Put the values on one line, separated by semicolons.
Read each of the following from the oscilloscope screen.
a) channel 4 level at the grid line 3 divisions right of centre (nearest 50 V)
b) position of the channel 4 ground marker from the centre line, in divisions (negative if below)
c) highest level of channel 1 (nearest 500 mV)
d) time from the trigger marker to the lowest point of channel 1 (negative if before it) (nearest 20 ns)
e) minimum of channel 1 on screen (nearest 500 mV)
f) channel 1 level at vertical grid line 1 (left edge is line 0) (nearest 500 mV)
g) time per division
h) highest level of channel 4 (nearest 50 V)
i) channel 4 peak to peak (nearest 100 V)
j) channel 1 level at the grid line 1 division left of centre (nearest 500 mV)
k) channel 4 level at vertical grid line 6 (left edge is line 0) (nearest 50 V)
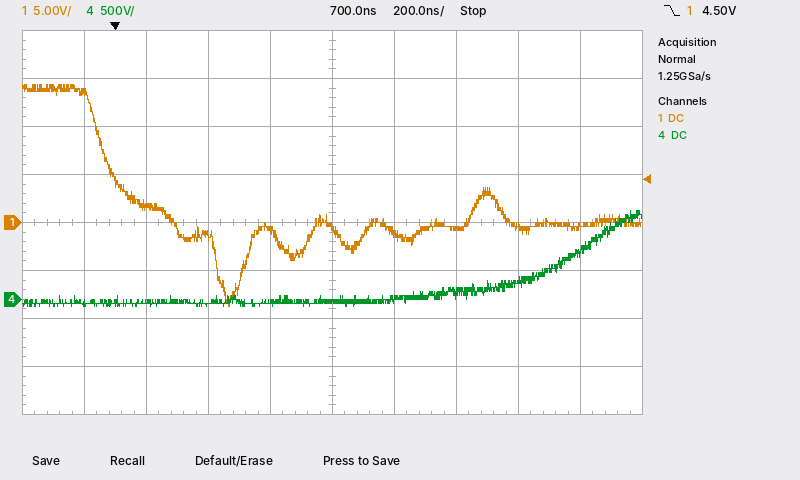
200 V; -1.6 div; 14.5 V; +360 ns; -9.0 V; 13.5 V; 200 ns; 900 V; 1.00 kV; -1.0 V; 0 V
